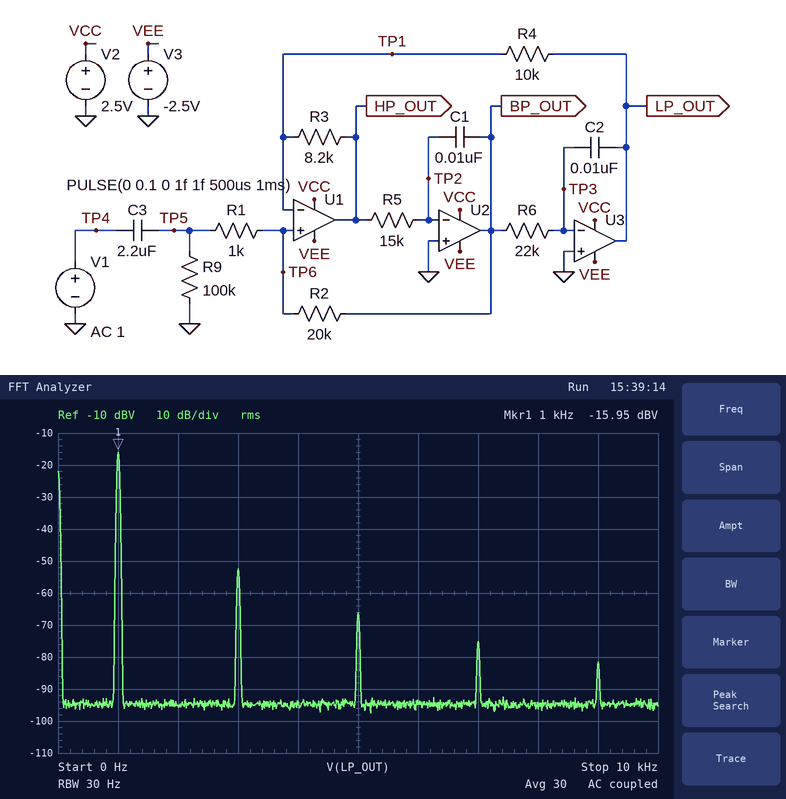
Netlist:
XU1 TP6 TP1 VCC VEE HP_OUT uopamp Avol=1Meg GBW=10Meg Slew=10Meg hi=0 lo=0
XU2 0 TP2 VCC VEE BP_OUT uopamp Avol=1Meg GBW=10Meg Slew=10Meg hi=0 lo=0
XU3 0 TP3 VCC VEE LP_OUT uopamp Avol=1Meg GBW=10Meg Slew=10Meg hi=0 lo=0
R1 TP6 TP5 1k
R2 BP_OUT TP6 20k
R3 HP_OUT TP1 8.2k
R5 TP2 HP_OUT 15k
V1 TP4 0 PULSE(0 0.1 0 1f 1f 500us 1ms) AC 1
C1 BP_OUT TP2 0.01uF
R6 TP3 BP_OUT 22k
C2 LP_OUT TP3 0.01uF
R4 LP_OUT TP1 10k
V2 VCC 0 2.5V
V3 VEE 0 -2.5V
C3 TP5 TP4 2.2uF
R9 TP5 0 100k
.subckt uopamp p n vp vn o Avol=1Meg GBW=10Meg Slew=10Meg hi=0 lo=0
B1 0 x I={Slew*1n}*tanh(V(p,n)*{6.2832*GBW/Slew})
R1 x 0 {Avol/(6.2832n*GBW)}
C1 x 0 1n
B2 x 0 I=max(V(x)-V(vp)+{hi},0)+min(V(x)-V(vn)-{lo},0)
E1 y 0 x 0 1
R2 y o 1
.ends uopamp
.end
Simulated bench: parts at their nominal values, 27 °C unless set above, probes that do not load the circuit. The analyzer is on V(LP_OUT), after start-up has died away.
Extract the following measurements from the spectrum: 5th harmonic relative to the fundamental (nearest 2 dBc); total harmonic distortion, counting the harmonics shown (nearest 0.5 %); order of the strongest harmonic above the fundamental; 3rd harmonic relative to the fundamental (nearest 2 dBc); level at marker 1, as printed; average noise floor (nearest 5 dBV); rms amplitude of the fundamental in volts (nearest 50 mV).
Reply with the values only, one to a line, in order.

-50 dBc
1.5 %
3
-36 dBc
-15.95 dBV
-95 dBV
150 mV
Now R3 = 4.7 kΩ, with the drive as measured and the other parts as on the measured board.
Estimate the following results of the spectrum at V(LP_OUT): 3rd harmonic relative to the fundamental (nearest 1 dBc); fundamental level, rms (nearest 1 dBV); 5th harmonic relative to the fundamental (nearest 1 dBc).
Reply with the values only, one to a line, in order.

-32 dBc
-22 dBV
-46 dBc
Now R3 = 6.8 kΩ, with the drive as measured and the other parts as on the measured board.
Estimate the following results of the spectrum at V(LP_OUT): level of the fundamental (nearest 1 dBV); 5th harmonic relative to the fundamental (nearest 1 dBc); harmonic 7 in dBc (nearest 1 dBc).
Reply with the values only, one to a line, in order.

-19 dBV
-48 dBc
-57 dBc
